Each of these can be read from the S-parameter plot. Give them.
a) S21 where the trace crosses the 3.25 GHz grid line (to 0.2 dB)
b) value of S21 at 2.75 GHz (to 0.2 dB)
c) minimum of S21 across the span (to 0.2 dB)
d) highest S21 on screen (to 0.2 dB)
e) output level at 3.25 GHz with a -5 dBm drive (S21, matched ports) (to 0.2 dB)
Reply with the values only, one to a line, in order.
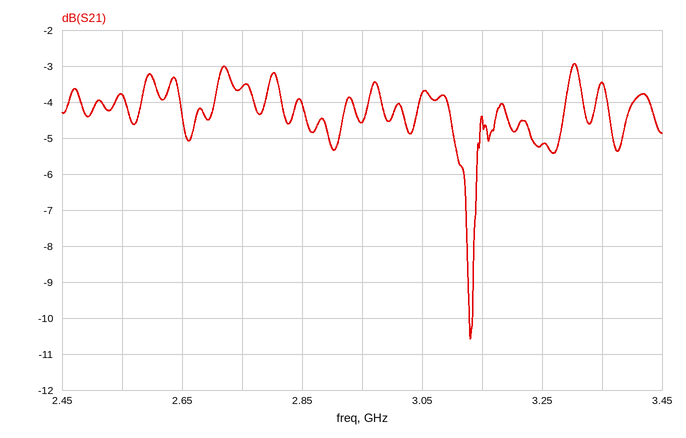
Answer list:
-5.2 dB
-3.6 dB
-10.6 dB
-3.0 dB
-10.2 dBm
